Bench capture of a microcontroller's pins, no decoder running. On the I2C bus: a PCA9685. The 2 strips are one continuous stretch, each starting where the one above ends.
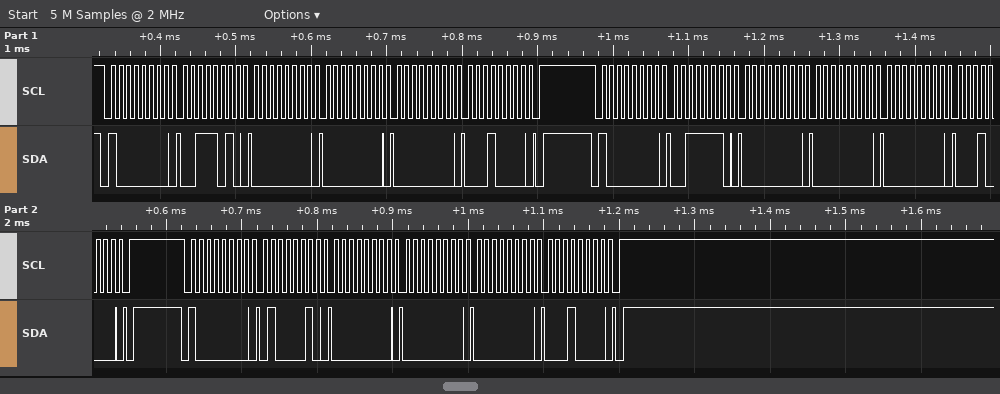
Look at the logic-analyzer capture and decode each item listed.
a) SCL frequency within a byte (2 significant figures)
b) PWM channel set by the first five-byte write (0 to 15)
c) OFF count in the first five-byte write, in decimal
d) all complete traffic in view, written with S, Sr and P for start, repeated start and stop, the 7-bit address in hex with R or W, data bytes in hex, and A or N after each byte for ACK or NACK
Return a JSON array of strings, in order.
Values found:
["100 kHz", "13", "4096", "S 40W A 3A A 00 A 00 A 00 A 10 A P S 40W A 3E A 00 A 00 A 00 A 10 A P S 40W A 42 A 00 A 00 A 00 A 10 A P"]
